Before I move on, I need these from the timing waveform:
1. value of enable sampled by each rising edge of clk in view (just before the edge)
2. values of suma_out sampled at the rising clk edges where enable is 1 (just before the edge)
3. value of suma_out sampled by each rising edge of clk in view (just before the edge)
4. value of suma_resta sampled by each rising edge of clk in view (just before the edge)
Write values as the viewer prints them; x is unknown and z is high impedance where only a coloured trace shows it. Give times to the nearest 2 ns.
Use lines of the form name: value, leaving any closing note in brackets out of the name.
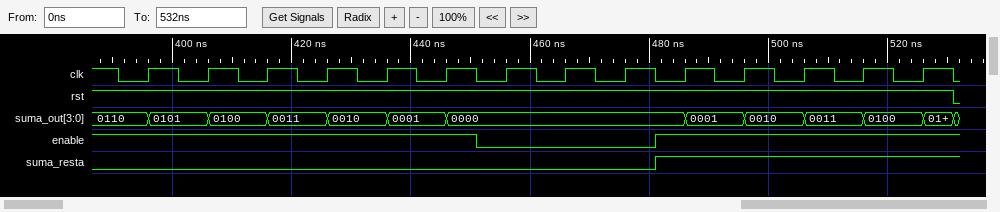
value of enable sampled by each rising edge of clk in view: 1 1 1 1 1 1 0 0 0 1 1 1 1 1
values of suma_out sampled at the rising clk edges where enable is 1: 0110, 0101, 0100, 0011, 0010, 0001, 0000, 0001, 0010, 0011, 0100
value of suma_out sampled by each rising edge of clk in view: 0110, 0101, 0100, 0011, 0010, 0001, 0000, 0000, 0000, 0000, 0001, 0010, 0011, 0100
value of suma_resta sampled by each rising edge of clk in view: 0 0 0 0 0 0 0 0 0 1 1 1 1 1
